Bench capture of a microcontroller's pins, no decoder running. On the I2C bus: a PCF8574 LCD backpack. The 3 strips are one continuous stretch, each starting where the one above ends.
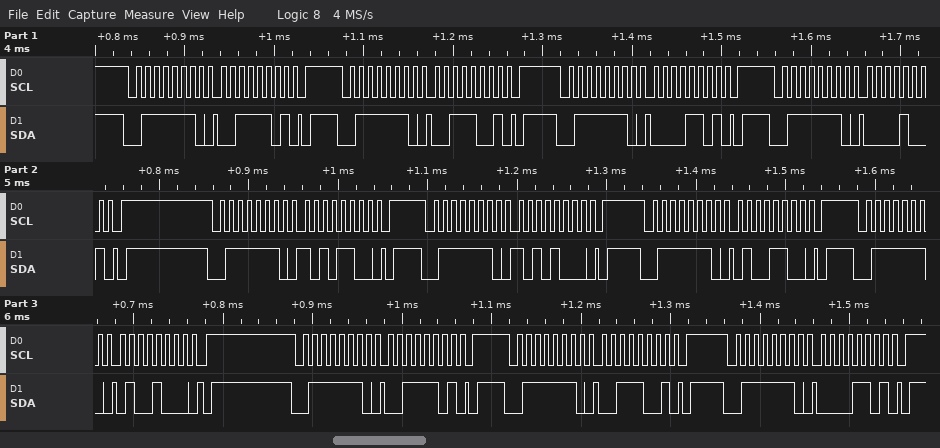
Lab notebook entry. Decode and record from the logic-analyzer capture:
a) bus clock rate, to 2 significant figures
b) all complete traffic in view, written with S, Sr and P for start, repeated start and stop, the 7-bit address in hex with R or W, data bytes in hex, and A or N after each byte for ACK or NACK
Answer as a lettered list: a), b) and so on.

a) 100 kHz
b) S 3FW A 3D A P S 3FW A 39 A P S 3FW A 0D A P S 3FW A 09 A P S 3FW A AC A P S 3FW A A8 A P S 3FW A 4C A P S 3FW A 48 A P S 3FW A 3D A P S 3FW A 39 A P S 3FW A 0D A P
